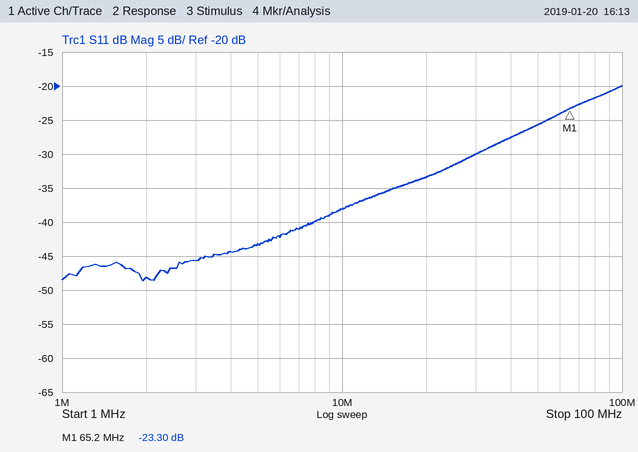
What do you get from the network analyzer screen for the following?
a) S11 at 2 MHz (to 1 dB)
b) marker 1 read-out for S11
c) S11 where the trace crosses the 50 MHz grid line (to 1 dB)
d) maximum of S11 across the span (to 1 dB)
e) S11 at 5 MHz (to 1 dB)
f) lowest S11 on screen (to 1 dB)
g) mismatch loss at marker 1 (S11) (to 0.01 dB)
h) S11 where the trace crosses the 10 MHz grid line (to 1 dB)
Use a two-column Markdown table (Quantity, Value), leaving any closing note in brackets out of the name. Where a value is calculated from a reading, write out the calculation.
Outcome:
| Quantity | Value |
|---|---|
| S11 at 2 MHz | -48 dB |
| marker 1 read-out for S11 | -23.30 dB |
| S11 where the trace crosses the 50 MHz grid line | -26 dB |
| maximum of S11 across the span | -20 dB |
| S11 at 5 MHz | -43 dB |
| lowest S11 on screen | -49 dB |
| mismatch loss at marker 1 (S11) | −10 log10(1 − 10^(-23.3/10)) ≈ 0.02 dB |
| S11 where the trace crosses the 10 MHz grid line | -38 dB |
